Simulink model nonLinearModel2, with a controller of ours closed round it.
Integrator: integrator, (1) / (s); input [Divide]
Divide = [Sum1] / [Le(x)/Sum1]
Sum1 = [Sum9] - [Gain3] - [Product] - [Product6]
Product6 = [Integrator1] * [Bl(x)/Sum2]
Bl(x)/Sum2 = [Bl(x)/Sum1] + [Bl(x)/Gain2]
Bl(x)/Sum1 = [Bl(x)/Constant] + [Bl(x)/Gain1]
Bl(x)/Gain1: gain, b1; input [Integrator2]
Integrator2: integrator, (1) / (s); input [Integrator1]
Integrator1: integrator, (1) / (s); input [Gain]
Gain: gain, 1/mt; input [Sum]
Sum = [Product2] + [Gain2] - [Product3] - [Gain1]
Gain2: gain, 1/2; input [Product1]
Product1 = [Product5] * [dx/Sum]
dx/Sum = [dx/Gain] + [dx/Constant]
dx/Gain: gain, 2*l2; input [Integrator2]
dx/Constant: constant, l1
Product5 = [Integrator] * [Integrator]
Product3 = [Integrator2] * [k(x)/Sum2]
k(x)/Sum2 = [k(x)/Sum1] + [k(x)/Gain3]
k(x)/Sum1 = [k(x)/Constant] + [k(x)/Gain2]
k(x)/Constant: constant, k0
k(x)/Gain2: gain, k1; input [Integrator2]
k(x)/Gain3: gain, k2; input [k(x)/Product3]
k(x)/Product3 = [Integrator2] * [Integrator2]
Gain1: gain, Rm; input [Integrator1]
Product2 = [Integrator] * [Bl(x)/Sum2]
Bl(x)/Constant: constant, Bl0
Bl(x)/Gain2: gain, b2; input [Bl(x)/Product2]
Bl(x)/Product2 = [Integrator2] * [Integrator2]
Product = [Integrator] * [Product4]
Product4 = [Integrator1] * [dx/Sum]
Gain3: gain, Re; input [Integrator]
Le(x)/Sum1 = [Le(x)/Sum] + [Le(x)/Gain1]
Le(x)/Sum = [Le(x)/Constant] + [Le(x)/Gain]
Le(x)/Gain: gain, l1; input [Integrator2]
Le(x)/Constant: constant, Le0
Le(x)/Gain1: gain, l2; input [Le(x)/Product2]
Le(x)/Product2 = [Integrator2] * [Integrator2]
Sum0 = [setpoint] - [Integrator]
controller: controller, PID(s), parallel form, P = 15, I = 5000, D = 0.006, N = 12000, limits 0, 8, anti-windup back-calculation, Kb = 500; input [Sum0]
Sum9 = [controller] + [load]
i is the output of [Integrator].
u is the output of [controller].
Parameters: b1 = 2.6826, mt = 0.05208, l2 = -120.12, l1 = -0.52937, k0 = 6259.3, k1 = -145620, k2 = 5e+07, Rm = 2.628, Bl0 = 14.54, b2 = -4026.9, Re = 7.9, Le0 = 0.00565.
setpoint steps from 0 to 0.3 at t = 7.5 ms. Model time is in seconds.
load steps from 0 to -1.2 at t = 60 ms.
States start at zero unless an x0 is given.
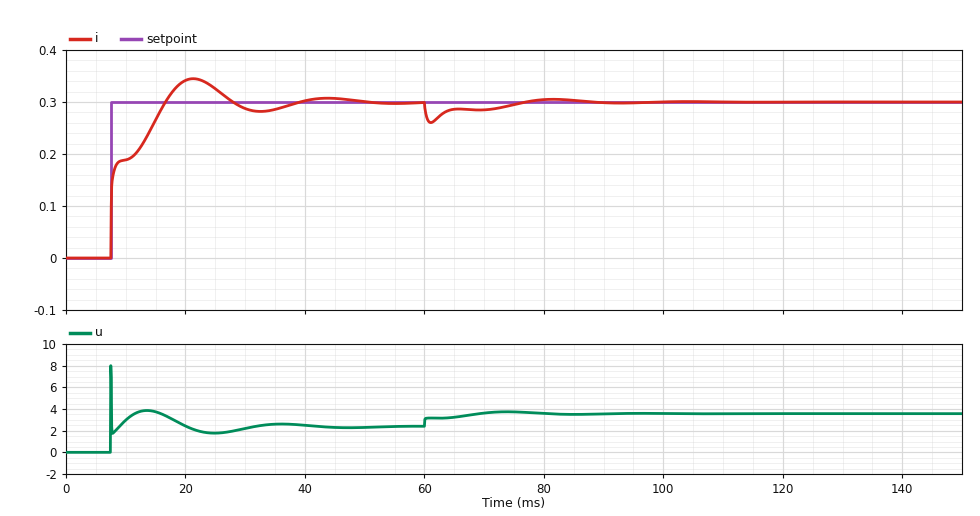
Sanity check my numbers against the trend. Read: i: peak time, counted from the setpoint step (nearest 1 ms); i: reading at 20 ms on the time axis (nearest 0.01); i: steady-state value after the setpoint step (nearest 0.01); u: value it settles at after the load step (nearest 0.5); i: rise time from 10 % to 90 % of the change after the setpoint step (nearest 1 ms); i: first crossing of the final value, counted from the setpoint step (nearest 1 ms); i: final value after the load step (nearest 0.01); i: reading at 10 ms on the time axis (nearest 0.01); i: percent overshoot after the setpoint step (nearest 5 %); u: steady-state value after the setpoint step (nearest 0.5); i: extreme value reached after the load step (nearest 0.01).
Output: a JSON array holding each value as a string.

["14 ms", "0.34", "0.30", "3.5", "8 ms", "9 ms", "0.30", "0.19", "15 %", "2.5", "0.26"]
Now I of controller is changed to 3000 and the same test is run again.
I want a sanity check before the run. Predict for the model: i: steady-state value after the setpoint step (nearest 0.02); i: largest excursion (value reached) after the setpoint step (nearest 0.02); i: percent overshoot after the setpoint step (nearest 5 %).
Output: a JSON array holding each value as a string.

["0.30", "0.32", "10 %"]
